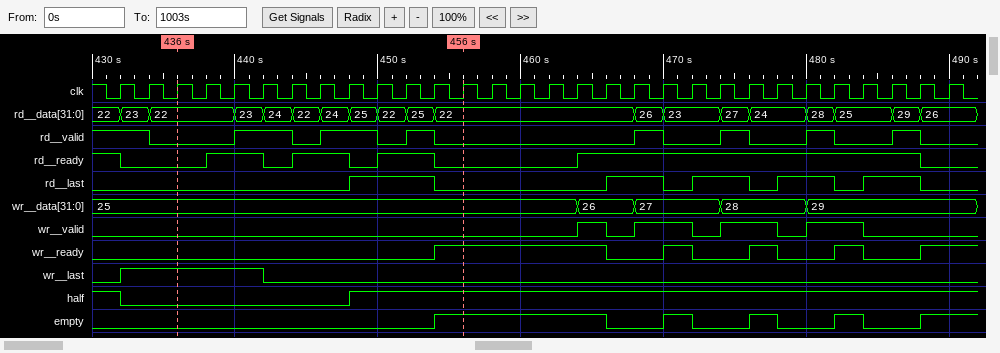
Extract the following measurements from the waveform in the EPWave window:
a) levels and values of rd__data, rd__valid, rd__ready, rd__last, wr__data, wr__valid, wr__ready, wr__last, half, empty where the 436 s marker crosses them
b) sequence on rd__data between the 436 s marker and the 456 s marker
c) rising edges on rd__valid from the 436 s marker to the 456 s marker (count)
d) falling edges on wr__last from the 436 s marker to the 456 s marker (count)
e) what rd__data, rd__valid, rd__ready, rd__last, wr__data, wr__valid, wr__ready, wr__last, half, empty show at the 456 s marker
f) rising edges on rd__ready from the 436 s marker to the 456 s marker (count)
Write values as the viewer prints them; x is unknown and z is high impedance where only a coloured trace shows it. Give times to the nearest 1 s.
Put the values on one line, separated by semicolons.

rd__data=22, rd__valid=0, rd__ready=0, rd__last=0, wr__data=25, wr__valid=0, wr__ready=0, wr__last=1, half=0, empty=0; 22, 23, 24, 22, 24, 25, 22, 25, 22; 3; 1; rd__data=22, rd__valid=0, rd__ready=0, rd__last=0, wr__data=25, wr__valid=0, wr__ready=1, wr__last=0, half=1, empty=1; 3
